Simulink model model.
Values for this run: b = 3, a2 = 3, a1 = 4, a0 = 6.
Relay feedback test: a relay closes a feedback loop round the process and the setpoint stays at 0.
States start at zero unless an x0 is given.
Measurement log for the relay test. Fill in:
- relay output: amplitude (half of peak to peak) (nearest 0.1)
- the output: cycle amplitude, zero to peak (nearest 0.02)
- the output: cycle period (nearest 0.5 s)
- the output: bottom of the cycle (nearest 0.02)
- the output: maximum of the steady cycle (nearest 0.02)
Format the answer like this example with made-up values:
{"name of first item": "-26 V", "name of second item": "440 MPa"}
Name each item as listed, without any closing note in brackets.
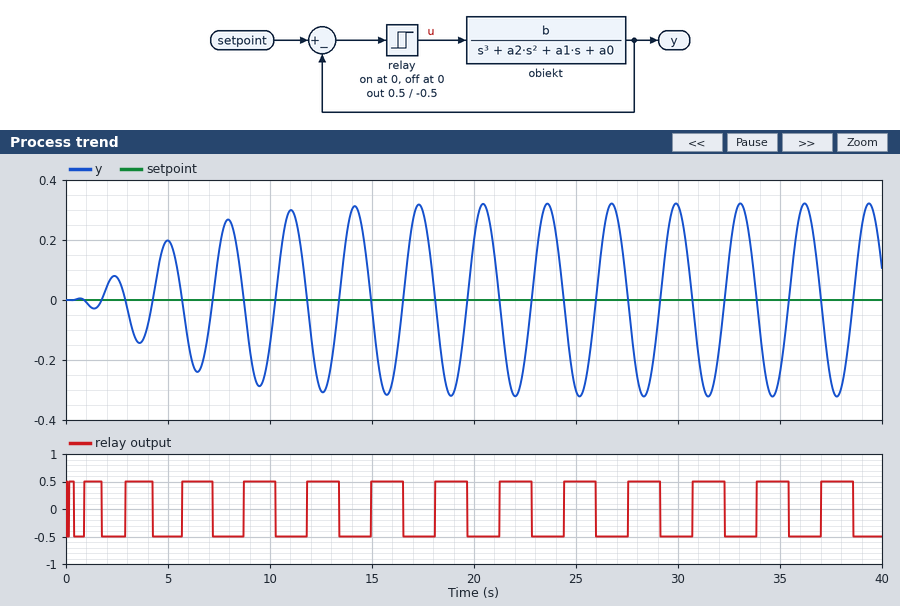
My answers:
{"relay output: amplitude (half of peak to peak)": "0.5", "the output: cycle amplitude, zero to peak": "0.32", "the output: cycle period": "3.0 s", "the output: bottom of the cycle": "-0.32", "the output: maximum of the steady cycle": "0.32"}
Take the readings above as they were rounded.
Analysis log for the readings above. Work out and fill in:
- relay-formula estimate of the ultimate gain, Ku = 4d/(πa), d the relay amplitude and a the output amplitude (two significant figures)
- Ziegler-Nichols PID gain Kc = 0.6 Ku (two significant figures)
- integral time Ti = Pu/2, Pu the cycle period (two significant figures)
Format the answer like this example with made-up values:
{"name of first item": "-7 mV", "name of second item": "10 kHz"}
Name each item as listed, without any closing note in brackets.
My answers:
{"relay-formula estimate of the ultimate gain, Ku = 4d/(πa), d the relay amplitude and a the output amplitude": "2.0", "Ziegler-Nichols PID gain Kc = 0.6 Ku": "1.2", "integral time Ti = Pu/2, Pu the cycle period": "1.5 s"}
